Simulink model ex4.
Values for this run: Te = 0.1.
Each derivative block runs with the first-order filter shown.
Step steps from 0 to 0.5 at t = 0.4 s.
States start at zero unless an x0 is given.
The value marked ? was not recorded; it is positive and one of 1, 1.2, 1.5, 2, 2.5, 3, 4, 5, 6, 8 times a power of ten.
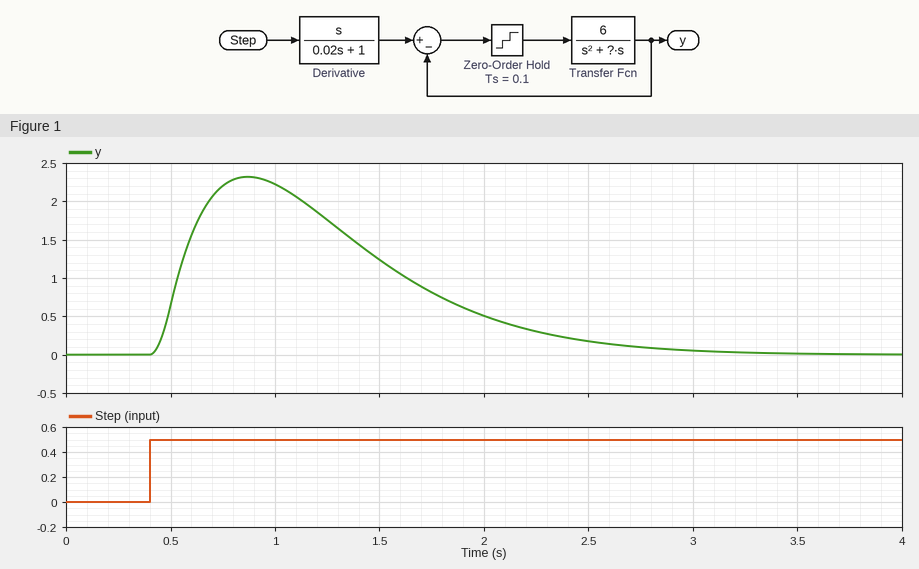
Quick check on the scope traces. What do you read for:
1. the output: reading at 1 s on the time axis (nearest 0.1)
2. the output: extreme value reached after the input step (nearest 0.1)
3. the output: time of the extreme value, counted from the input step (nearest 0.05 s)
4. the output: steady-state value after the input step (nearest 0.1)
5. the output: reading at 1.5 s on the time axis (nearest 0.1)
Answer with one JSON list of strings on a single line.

["2.2", "2.3", "0.45 s", "0.0", "1.2"]
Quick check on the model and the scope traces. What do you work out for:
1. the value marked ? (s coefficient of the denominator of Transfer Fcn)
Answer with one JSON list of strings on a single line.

["5"]
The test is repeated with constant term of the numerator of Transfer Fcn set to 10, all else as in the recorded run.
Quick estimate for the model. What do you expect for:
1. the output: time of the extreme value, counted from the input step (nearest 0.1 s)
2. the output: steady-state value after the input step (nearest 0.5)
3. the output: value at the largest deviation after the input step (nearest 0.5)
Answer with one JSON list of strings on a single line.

["0.4 s", "0.0", "3.5"]
